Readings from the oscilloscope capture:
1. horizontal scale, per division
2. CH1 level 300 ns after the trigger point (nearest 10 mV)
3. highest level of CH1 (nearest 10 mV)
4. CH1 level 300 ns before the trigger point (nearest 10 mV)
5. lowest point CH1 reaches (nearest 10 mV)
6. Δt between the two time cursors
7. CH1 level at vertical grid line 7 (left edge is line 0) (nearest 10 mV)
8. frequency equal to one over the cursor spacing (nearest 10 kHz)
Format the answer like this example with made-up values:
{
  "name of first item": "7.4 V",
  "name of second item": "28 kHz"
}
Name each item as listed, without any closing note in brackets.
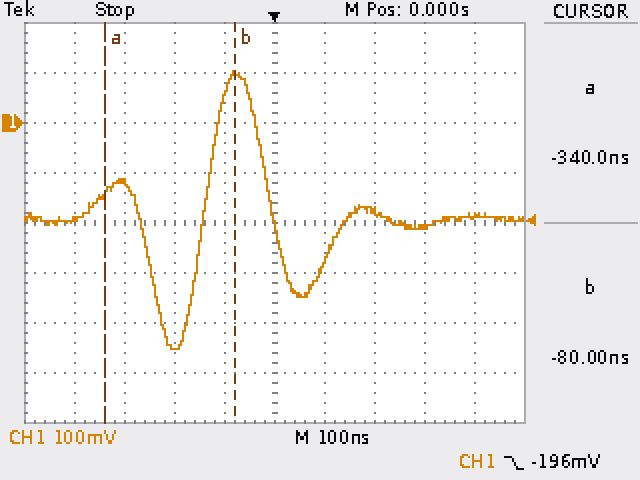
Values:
{
  "horizontal scale, per division": "100 ns",
  "CH1 level 300 ns after the trigger point": "-210 mV",
  "highest level of CH1": "100 mV",
  "CH1 level 300 ns before the trigger point": "-120 mV",
  "lowest point CH1 reaches": "-450 mV",
  "Δt between the two time cursors": "260 ns",
  "CH1 level at vertical grid line 7 (left edge is line 0)": "-180 mV",
  "frequency equal to one over the cursor spacing": "3.85 MHz"
}
